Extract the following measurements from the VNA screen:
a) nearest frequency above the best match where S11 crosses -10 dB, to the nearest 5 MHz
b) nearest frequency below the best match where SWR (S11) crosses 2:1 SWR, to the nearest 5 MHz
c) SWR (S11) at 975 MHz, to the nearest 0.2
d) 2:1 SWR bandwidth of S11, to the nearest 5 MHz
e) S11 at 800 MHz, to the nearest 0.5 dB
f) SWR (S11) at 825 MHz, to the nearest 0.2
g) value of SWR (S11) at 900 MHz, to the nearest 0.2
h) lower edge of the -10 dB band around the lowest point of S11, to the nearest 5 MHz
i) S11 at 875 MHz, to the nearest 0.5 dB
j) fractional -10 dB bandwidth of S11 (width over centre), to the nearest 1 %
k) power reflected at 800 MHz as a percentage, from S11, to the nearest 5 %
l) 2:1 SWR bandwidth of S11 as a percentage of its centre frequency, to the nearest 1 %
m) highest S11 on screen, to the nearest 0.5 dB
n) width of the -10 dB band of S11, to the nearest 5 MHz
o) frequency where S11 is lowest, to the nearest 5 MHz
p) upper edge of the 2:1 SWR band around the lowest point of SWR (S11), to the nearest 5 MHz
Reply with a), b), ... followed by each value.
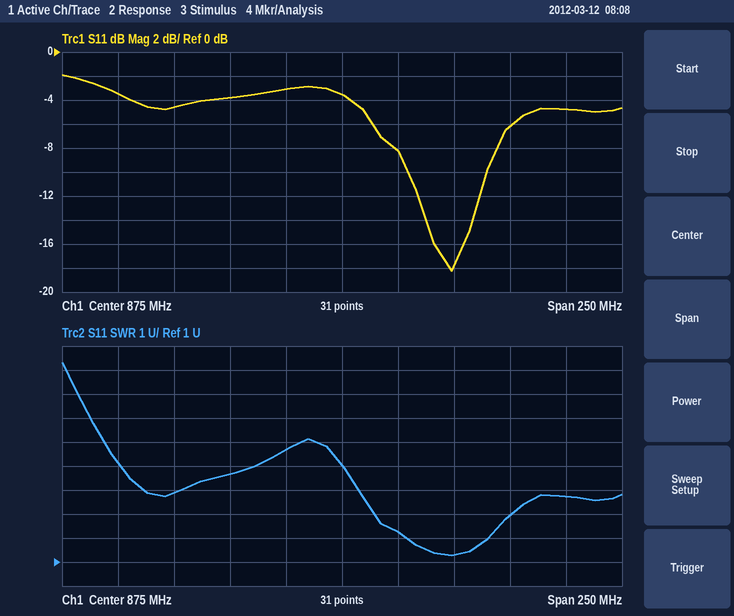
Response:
a) 940 MHz
b) 905 MHz
c) 3.8
d) 35 MHz
e) -4.5 dB
f) 4.6
g) 2.2
h) 905 MHz
i) -3.5 dB
j) 4 %
k) 35 %
l) 4 %
m) -2.0 dB
n) 35 MHz
o) 925 MHz
p) 940 MHz
